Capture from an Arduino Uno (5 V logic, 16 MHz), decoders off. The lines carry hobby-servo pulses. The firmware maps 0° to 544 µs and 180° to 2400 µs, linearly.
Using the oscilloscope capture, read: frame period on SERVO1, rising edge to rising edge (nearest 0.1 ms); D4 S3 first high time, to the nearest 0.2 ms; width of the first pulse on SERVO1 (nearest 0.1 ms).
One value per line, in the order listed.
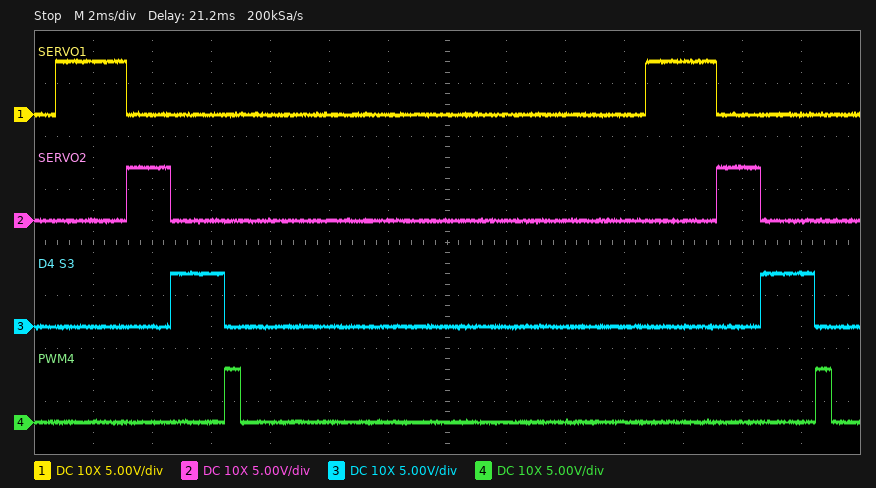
20.0 ms
1.8 ms
2.4 ms
